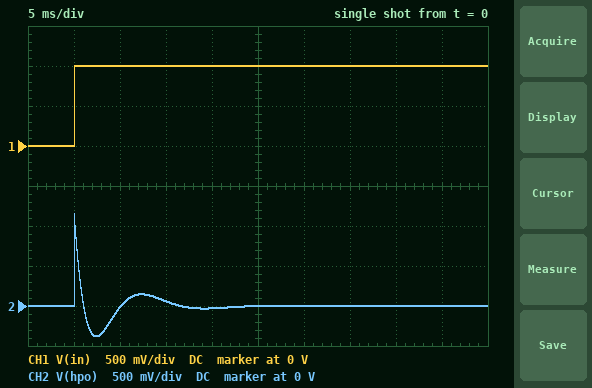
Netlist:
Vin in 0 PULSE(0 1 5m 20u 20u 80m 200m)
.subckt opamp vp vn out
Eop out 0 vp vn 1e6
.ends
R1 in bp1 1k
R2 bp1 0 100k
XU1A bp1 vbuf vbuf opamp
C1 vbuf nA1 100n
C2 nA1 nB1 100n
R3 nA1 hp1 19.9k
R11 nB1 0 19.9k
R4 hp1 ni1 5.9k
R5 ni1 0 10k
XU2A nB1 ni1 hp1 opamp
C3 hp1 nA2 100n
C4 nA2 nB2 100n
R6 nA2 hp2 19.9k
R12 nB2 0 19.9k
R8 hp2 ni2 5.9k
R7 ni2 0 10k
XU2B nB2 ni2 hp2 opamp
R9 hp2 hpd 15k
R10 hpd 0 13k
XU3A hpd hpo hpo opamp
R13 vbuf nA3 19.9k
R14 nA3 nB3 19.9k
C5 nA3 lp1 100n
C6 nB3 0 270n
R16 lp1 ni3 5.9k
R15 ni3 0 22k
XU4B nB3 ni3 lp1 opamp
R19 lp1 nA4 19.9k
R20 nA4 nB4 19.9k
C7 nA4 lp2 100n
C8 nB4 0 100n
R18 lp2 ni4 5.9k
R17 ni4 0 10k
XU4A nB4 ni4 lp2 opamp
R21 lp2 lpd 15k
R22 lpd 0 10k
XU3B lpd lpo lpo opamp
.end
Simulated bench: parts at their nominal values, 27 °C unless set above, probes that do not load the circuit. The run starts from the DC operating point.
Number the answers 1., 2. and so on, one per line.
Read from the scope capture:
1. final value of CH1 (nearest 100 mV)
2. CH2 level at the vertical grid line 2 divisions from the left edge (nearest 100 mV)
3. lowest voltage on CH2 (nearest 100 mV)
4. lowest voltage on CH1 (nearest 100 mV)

1. 1.0 V
2. 0 V
3. -400 mV
4. 0 V
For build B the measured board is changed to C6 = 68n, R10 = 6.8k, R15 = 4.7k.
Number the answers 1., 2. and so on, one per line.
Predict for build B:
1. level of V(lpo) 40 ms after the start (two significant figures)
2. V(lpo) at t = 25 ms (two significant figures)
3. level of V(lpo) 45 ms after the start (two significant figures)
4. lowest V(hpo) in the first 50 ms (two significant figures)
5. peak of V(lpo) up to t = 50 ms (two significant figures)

1. 1.2 V
2. 1.7 V
3. 1.6 V
4. -260 mV
5. 2.1 V
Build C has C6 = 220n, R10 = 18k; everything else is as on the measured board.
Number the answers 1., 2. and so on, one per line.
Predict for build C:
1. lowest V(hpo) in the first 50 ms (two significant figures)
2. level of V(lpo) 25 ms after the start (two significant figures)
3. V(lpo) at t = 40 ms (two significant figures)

1. -450 mV
2. 720 mV
3. 790 mV
